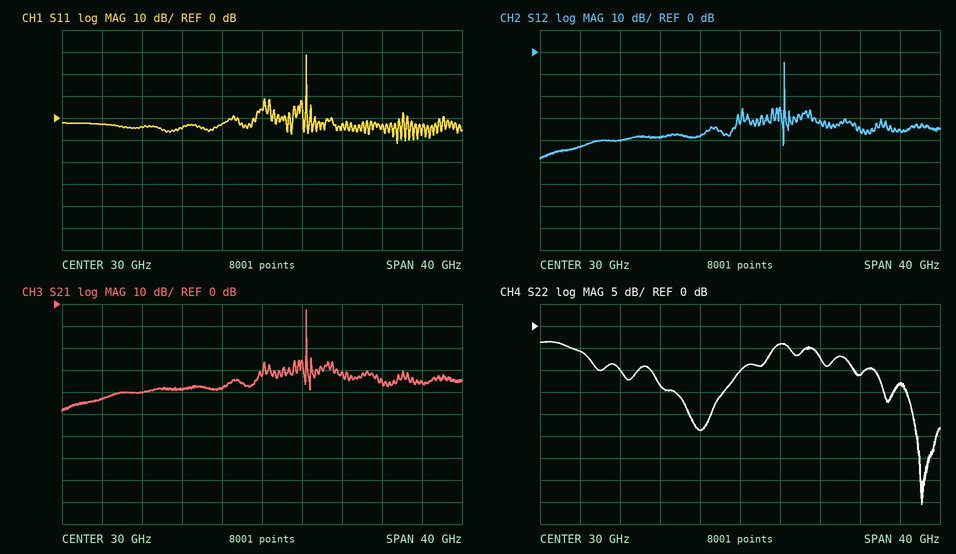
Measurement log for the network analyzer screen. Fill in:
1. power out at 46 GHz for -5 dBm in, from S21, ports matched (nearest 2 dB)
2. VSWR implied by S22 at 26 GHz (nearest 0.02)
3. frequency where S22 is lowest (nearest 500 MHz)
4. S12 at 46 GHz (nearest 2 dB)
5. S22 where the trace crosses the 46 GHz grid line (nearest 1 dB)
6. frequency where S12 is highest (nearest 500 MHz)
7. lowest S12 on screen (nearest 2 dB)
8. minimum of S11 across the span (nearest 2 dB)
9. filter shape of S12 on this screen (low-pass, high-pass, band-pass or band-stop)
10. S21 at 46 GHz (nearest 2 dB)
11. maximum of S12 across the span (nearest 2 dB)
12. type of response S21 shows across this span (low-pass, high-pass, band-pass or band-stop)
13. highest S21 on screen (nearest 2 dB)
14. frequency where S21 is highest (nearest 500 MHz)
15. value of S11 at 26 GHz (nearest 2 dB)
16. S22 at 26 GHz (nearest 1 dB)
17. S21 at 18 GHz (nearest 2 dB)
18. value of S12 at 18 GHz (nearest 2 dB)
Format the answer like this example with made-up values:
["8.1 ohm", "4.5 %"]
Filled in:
["-40 dBm", "1.14", "48.0 GHz", "-36 dB", "-13 dB", "34.5 GHz", "-48 dB", "-12 dB", "band-pass", "-36 dB", "-4 dB", "band-pass", "-2 dB", "34.5 GHz", "-2 dB", "-24 dB", "-40 dB", "-40 dB"]
